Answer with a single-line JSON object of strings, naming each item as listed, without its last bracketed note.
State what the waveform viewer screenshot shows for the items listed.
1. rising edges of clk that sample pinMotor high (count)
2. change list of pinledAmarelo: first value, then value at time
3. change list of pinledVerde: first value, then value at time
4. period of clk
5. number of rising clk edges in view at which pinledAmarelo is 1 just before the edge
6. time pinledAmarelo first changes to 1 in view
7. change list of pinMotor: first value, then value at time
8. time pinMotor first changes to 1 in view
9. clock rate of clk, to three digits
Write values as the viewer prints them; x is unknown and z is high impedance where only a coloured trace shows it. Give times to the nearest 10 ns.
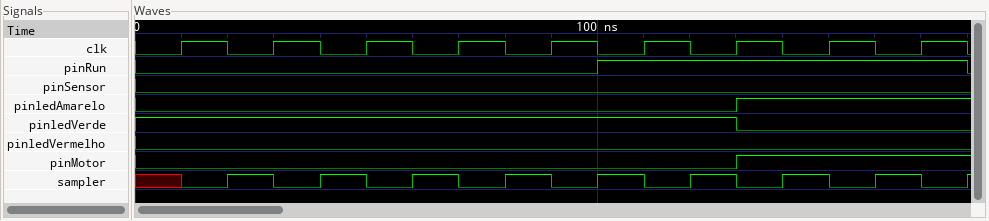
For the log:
{"rising edges of clk that sample pinMotor high": "2", "change list of pinledAmarelo: first value, then value at time": "0, 1 at 130 ns", "change list of pinledVerde: first value, then value at time": "1, 0 at 130 ns", "period of clk": "20 ns", "number of rising clk edges in view at which pinledAmarelo is 1 just before the edge": "2", "time pinledAmarelo first changes to 1 in view": "130 ns", "change list of pinMotor: first value, then value at time": "0, 1 at 130 ns", "time pinMotor first changes to 1 in view": "130 ns", "clock rate of clk, to three digits": "50.0 MHz"}
